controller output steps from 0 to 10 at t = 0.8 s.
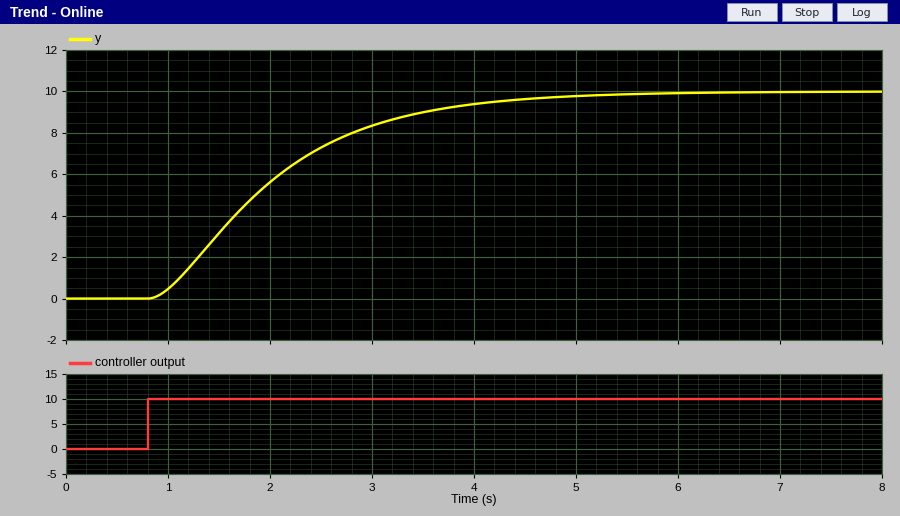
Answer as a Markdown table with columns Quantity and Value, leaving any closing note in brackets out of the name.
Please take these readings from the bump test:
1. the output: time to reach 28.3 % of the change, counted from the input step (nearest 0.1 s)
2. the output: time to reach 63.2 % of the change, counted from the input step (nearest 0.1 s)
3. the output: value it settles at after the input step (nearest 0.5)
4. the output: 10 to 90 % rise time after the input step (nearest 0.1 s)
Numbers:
| Quantity | Value |
|---|---|
| the output: time to reach 28.3 % of the change, counted from the input step | 0.6 s |
| the output: time to reach 63.2 % of the change, counted from the input step | 1.4 s |
| the output: value it settles at after the input step | 10.0 |
| the output: 10 to 90 % rise time after the input step | 2.4 s |
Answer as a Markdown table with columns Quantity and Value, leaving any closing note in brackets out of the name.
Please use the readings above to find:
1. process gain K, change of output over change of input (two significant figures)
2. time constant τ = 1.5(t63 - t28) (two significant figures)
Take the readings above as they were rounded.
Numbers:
| Quantity | Value |
|---|---|
| process gain K, change of output over change of input | 1.0 |
| time constant τ = 1.5(t63 - t28) | 1.2 s |
